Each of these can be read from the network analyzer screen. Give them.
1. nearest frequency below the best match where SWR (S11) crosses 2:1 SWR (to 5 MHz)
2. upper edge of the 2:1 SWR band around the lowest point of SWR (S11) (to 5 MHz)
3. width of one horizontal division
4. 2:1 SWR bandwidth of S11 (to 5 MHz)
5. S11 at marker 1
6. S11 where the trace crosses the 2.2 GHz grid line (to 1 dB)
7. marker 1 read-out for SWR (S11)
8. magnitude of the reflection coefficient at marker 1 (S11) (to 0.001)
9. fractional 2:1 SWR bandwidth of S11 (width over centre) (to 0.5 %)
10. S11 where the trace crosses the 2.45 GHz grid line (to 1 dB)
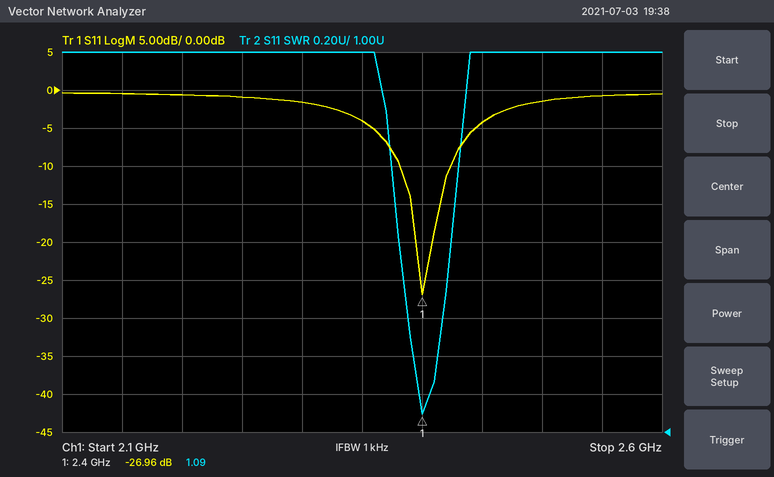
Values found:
2.380 GHz
2.425 GHz
50 MHz
45 MHz
-26.96 dB
-1 dB
1.09
0.045
2.0 %
-4 dB
